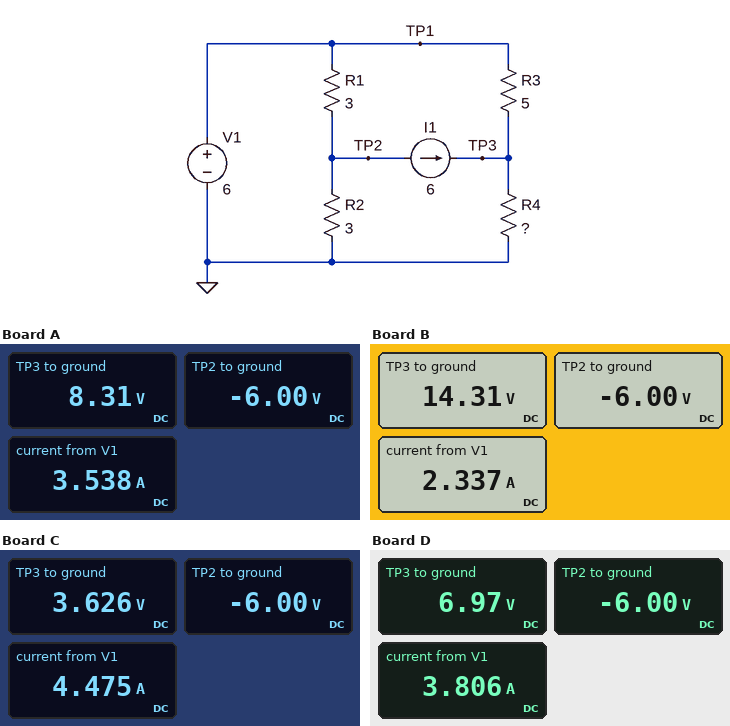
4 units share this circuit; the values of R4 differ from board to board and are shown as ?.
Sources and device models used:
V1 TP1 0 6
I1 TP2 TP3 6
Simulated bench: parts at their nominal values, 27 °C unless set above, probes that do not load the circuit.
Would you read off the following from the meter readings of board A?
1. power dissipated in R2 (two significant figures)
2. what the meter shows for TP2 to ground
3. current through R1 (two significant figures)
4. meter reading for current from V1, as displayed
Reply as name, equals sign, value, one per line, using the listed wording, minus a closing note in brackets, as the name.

power dissipated in R2 = 12 W
what the meter shows for TP2 to ground = -6.00 V
current through R1 = 4.0 A
meter reading for current from V1, as displayed = 3.538 A
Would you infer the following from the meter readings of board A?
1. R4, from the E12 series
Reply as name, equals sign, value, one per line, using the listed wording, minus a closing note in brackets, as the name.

R4, from the E12 series = 1.5 Ω
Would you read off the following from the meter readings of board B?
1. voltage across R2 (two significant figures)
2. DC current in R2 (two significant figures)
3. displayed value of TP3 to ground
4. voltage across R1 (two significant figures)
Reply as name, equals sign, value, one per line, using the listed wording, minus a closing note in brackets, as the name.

voltage across R2 = 6.0 V
DC current in R2 = 2.0 A
displayed value of TP3 to ground = 14.31 V
voltage across R1 = 12 V
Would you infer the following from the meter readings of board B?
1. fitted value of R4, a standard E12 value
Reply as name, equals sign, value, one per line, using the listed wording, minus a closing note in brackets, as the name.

fitted value of R4, a standard E12 value = 3.3 Ω
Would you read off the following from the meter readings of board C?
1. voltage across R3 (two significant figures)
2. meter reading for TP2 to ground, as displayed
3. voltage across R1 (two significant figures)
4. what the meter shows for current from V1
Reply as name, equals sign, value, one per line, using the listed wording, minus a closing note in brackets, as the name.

voltage across R3 = 2.4 V
meter reading for TP2 to ground, as displayed = -6.00 V
voltage across R1 = 12 V
what the meter shows for current from V1 = 4.475 A
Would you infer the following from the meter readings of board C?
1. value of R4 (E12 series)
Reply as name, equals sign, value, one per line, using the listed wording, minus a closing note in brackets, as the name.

value of R4 = 0.56 Ω
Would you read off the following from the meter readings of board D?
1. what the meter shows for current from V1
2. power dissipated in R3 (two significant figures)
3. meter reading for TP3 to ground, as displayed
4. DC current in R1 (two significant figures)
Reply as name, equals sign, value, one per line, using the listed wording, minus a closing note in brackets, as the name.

what the meter shows for current from V1 = 3.806 A
power dissipated in R3 = 190 mW
meter reading for TP3 to ground, as displayed = 6.97 V
DC current in R1 = 4.0 A
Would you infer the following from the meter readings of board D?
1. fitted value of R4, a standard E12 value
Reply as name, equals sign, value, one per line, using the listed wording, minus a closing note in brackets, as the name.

fitted value of R4, a standard E12 value = 1.2 Ω
